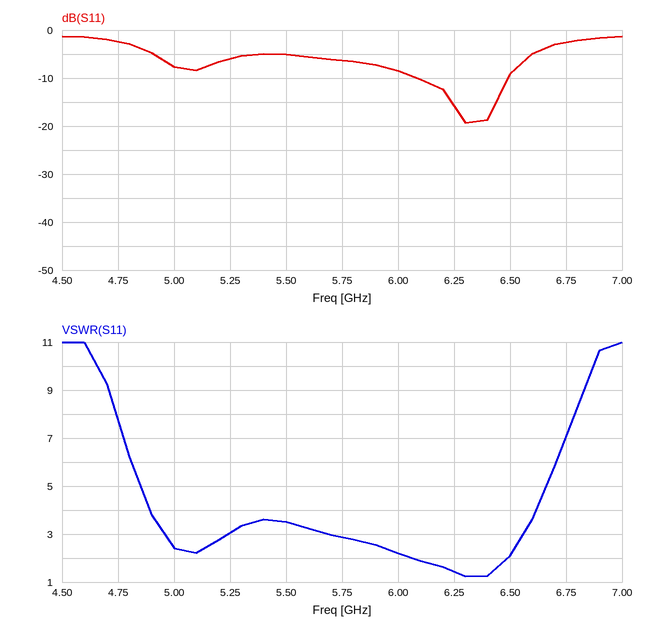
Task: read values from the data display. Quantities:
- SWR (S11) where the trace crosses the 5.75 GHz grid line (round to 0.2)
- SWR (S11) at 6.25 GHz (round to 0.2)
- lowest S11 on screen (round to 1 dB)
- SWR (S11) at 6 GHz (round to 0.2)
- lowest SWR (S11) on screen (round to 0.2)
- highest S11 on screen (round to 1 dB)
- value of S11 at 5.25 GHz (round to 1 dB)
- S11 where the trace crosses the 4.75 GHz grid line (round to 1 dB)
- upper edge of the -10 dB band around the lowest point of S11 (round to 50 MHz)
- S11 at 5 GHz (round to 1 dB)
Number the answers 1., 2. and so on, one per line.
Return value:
1. 2.8
2. 1.4
3. -19 dB
4. 2.2
5. 1.2
6. -1 dB
7. -6 dB
8. -2 dB
9. 6.50 GHz
10. -8 dB
